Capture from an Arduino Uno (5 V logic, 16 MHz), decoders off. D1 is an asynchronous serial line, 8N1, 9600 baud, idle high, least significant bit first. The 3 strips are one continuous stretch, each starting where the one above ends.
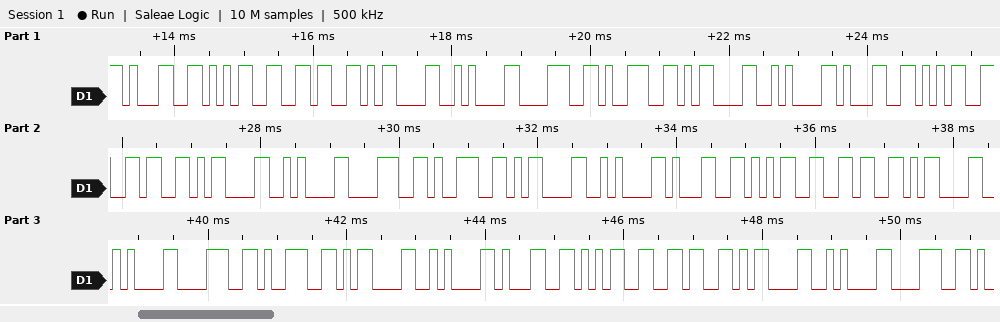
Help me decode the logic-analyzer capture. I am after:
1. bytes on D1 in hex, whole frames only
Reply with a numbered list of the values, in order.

1. 31 35 36 0D 0A 38 39 0D 0A 31 35 36 0D 0A 38 39 0D 0A 31 35 36 0D 0A 38 39 0D 0A 31 35 36 0D 0A 38
